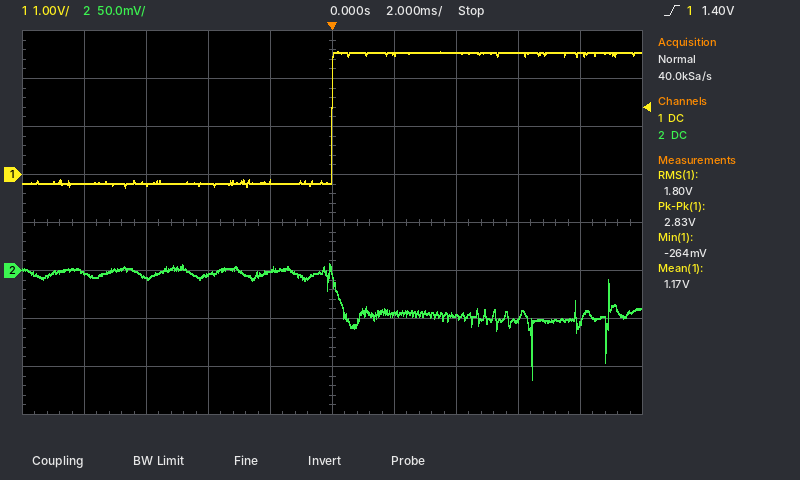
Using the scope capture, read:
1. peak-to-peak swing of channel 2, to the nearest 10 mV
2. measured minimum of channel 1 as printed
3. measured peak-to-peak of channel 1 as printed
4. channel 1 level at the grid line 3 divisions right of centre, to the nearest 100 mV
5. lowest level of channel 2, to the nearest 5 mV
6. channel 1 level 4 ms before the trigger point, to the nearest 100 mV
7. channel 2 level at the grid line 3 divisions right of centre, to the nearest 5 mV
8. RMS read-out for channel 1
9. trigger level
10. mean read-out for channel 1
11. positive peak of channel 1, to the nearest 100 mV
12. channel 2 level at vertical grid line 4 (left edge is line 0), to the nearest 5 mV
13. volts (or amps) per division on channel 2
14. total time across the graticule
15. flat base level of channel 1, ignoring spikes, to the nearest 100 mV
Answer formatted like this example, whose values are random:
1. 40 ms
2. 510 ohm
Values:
1. 120 mV
2. -264 mV
3. 2.83 V
4. 2.5 V
5. -115 mV
6. -200 mV
7. -50 mV
8. 1.80 V
9. 1.40 V
10. 1.17 V
11. 2.6 V
12. 0 mV
13. 50 mV
14. 20 ms
15. -200 mV
